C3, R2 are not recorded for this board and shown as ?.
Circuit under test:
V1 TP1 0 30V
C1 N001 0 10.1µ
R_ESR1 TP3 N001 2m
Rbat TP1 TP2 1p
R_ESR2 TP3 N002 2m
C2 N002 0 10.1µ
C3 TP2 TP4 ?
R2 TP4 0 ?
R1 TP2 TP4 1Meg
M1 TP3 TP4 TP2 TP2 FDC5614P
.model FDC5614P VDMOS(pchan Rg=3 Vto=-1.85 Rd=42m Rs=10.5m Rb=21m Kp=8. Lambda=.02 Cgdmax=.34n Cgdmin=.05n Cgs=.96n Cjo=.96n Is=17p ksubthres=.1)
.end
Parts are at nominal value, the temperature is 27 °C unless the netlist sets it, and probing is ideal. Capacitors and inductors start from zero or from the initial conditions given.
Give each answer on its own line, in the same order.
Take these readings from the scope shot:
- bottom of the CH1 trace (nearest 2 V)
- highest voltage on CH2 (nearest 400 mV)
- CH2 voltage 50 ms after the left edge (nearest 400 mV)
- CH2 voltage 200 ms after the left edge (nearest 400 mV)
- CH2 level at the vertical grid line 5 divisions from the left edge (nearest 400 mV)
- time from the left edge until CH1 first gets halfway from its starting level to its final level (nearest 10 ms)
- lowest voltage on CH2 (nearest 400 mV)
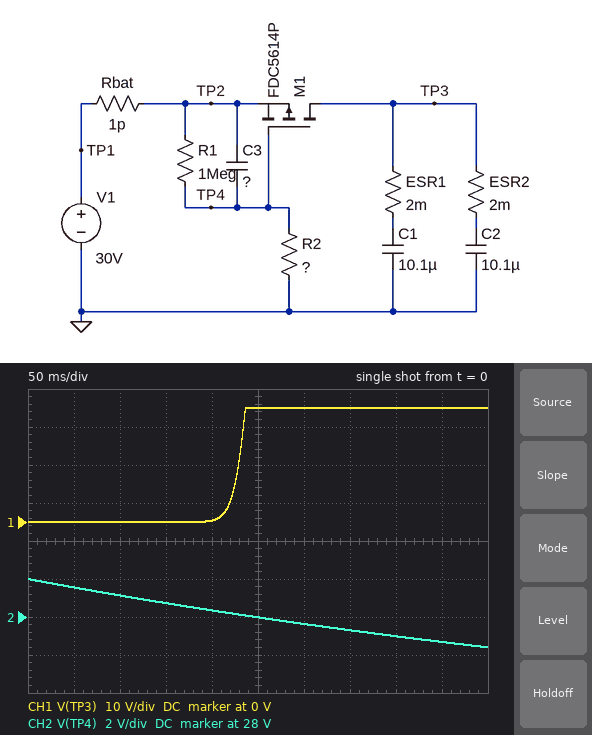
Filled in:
0 V
30.0 V
29.6 V
28.4 V
28.0 V
230 ms
26.4 V
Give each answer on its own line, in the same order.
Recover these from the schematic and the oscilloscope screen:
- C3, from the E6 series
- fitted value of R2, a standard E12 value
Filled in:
1.5 µF
2.2 MΩ
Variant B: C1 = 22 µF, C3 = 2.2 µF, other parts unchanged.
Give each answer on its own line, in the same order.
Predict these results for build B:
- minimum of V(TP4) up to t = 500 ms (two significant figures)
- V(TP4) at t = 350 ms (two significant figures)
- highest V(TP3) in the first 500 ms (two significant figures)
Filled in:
27 V
28 V
30 V
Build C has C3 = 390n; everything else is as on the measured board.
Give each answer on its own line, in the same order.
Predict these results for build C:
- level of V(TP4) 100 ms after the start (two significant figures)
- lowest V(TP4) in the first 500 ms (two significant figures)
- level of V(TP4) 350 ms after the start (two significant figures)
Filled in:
27 V
22 V
23 V
